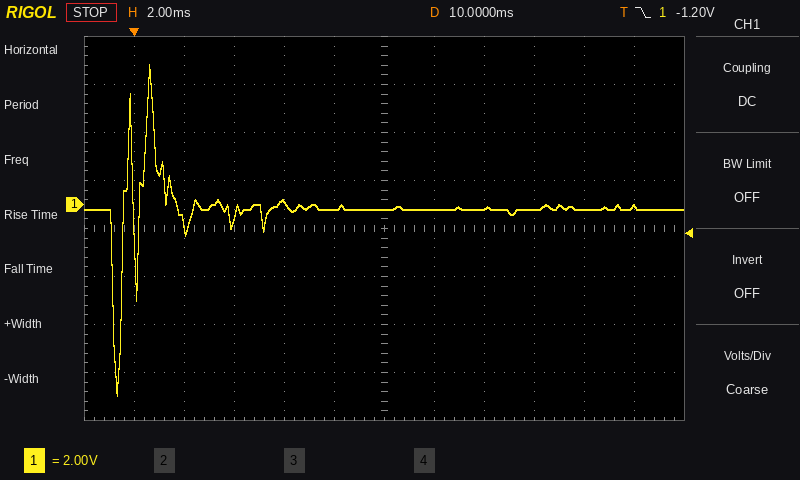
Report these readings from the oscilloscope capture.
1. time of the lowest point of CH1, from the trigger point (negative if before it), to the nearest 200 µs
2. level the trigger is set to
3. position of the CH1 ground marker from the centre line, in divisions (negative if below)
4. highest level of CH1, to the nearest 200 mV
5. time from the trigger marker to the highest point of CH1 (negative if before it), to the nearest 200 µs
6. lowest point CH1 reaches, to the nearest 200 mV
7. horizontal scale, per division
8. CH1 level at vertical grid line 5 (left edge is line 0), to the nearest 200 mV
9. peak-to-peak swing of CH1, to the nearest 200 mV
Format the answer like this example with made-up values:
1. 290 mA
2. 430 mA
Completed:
1. -600 µs
2. -1.20 V
3. +0.5 div
4. 5.8 V
5. +600 µs
6. -8.0 V
7. 2 ms
8. -200 mV
9. 13.8 V
